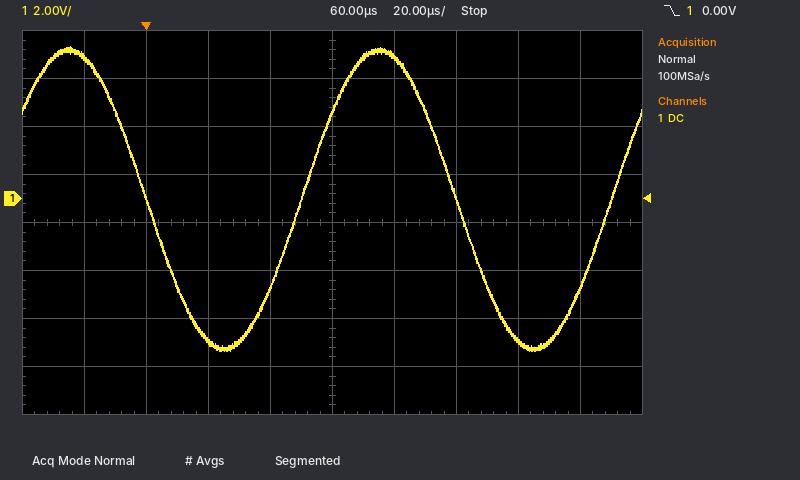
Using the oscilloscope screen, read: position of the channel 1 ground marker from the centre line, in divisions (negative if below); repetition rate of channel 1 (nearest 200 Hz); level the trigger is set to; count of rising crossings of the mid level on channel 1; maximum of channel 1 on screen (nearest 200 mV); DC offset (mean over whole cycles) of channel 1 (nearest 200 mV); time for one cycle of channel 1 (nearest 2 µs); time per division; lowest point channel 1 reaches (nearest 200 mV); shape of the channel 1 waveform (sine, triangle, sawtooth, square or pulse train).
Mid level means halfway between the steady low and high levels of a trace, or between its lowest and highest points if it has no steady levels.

+0.5 div
10.0 kHz
0.00 V
2
6.4 V
0.0 V
100 µs
20 µs
-6.4 V
sine
